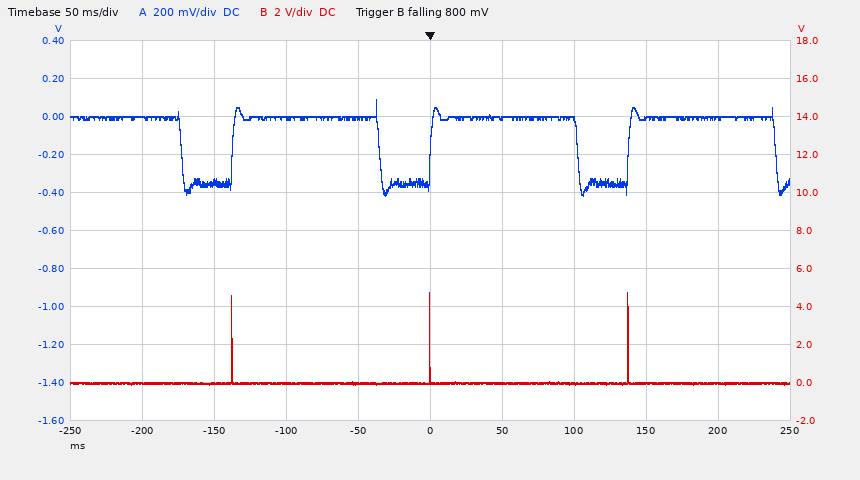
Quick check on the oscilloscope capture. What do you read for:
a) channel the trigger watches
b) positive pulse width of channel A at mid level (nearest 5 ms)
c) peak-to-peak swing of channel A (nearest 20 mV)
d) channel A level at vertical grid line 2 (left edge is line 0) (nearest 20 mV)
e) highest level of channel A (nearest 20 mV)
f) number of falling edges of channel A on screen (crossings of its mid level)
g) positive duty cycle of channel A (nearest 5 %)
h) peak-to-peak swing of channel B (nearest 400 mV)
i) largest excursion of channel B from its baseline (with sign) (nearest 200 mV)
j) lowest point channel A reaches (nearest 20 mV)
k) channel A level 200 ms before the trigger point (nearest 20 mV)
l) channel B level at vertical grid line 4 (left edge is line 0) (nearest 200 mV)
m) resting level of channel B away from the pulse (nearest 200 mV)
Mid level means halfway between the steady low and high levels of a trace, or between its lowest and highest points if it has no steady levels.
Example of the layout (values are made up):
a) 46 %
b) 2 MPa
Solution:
a) channel B
b) 100 ms
c) 500 mV
d) -340 mV
e) 80 mV
f) 4
g) 75 %
h) 4.8 V
i) +4.8 V
j) -420 mV
k) 0 mV
l) 0.0 V
m) 0.0 V
